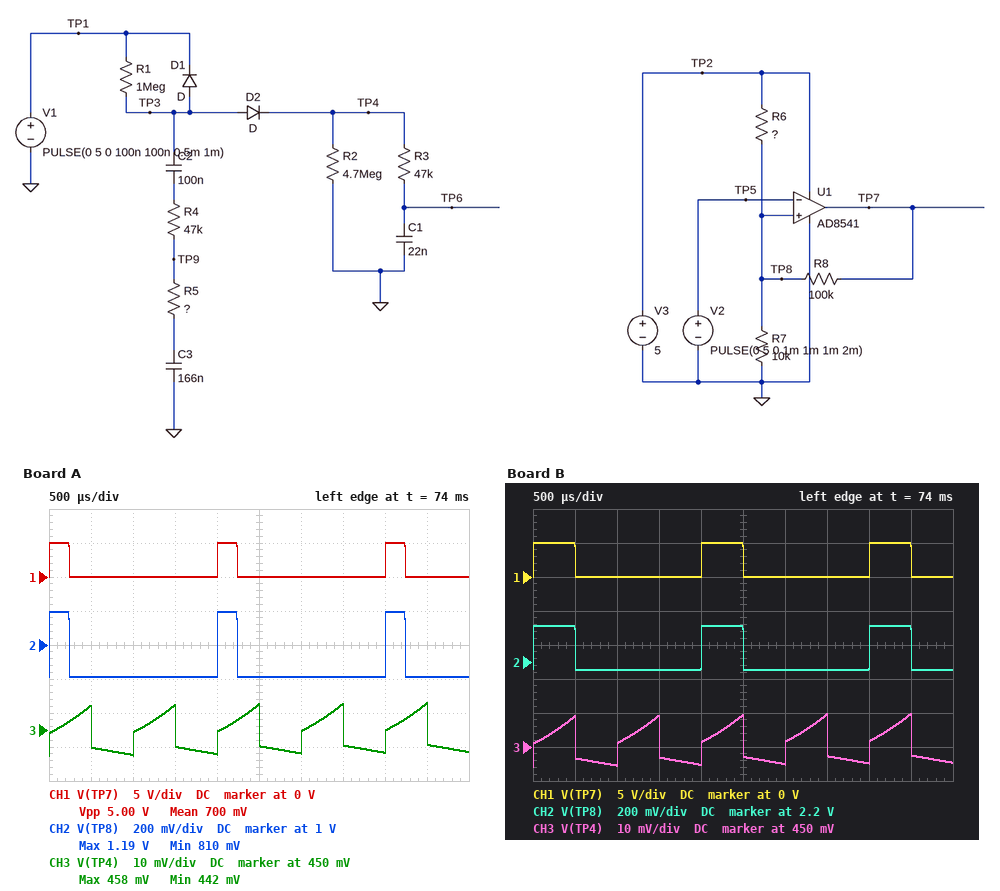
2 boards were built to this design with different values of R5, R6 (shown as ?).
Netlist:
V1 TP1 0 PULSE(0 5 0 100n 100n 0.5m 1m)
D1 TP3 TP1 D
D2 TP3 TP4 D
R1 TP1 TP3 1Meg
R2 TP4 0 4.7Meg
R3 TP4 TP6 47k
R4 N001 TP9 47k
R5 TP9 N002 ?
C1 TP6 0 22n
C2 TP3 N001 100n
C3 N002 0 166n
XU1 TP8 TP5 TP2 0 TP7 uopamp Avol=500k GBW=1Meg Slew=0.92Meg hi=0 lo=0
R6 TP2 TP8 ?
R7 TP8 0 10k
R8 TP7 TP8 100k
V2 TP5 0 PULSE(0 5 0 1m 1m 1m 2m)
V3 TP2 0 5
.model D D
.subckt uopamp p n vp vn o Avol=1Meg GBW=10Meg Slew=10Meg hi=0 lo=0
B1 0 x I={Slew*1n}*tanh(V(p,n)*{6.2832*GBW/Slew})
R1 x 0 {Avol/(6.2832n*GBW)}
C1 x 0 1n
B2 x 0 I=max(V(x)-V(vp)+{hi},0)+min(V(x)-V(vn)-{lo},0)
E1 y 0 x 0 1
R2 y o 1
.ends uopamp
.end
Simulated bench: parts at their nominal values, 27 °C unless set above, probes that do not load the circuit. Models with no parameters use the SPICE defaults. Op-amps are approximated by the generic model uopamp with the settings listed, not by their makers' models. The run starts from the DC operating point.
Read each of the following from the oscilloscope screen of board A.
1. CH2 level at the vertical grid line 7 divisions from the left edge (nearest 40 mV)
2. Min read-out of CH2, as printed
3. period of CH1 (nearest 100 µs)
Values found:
800 mV
810 mV
2.0 ms
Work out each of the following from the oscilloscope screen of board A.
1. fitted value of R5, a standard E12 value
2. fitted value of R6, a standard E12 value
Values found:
1.5 kΩ
47 kΩ
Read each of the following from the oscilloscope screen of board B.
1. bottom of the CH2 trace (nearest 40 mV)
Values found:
2.16 V
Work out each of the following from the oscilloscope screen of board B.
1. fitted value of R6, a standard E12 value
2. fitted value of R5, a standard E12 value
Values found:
12 kΩ
1.8 kΩ
